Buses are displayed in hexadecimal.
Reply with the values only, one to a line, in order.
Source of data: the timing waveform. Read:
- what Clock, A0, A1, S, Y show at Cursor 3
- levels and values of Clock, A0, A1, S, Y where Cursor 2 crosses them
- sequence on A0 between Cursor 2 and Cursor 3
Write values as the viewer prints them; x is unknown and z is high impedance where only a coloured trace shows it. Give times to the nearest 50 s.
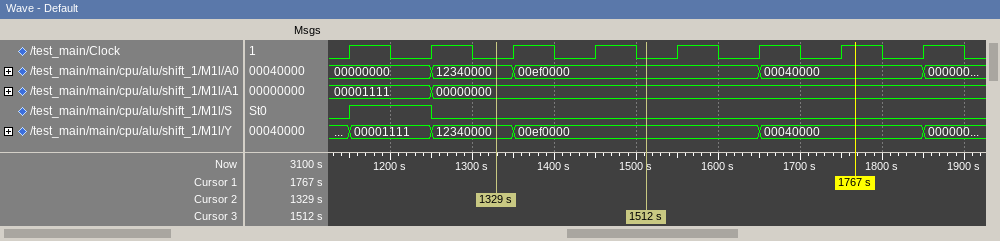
Clock=0, A0=00ef0000, A1=00000000, S=0, Y=00ef0000
Clock=0, A0=12340000, A1=00000000, S=0, Y=12340000
12340000, 00ef0000
